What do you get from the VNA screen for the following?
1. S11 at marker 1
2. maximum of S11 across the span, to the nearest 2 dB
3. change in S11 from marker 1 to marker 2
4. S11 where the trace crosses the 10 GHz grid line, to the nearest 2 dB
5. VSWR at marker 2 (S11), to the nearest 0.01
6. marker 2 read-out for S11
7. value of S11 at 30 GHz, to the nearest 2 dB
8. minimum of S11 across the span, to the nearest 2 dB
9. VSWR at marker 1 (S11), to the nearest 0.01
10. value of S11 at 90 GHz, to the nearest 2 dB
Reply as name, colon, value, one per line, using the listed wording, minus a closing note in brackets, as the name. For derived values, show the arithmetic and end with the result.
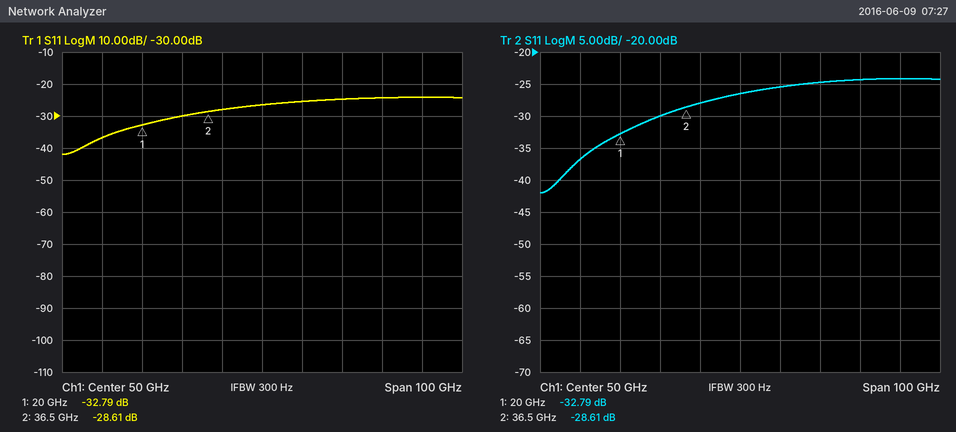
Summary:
S11 at marker 1: -32.79 dB
maximum of S11 across the span, to the nearest 2 dB: -24 dB
change in S11 from marker 1 to marker 2: -28.61 − (-32.79) = 4.18 dB
S11 where the trace crosses the 10 GHz grid line, to the nearest 2 dB: -36 dB
VSWR at marker 2 (S11), to the nearest 0.01: (1 + 0.0371)/(1 − 0.0371) ≈ 1.08
marker 2 read-out for S11: -28.61 dB
value of S11 at 30 GHz, to the nearest 2 dB: -30 dB
minimum of S11 across the span, to the nearest 2 dB: -42 dB
VSWR at marker 1 (S11), to the nearest 0.01: (1 + 0.0229)/(1 − 0.0229) ≈ 1.05
value of S11 at 90 GHz, to the nearest 2 dB: -24 dB
